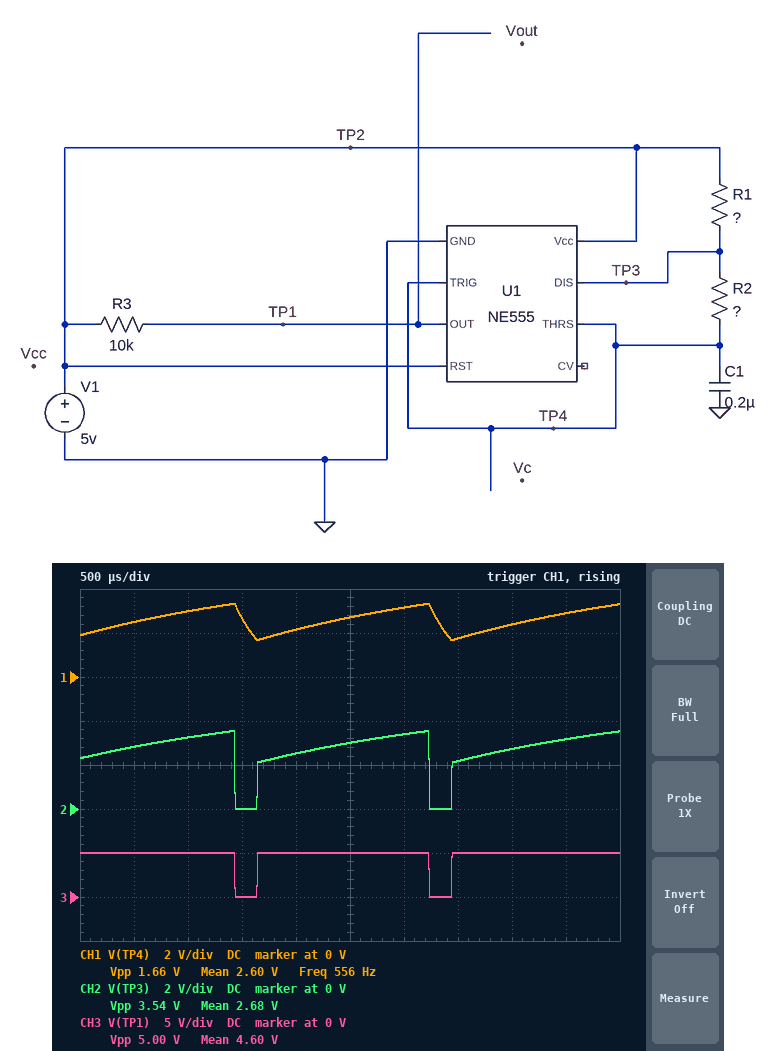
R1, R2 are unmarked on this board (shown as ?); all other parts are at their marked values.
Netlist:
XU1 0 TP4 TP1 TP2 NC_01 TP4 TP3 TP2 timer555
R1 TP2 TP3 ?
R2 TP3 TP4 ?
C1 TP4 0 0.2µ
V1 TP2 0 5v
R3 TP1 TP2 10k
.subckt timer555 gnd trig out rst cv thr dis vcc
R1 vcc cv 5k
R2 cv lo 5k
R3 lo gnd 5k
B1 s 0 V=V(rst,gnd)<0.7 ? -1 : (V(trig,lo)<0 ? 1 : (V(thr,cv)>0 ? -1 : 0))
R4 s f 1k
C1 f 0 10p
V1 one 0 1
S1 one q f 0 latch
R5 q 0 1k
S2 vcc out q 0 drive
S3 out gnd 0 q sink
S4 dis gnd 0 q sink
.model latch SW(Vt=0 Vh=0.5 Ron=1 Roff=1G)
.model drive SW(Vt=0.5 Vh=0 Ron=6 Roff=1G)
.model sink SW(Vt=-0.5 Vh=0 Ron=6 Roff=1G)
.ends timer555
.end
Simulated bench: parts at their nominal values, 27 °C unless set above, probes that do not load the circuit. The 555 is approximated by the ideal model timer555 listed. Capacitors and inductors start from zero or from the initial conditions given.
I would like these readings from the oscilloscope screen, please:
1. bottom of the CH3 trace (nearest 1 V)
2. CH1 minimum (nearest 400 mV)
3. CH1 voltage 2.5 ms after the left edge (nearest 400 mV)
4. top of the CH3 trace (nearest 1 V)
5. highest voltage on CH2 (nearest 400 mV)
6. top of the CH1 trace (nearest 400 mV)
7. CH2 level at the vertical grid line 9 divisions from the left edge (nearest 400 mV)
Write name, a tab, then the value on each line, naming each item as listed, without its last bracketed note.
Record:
bottom of the CH3 trace	0 V
CH1 minimum	1.6 V
CH1 voltage 2.5 ms after the left edge	2.8 V
top of the CH3 trace	5 V
highest voltage on CH2	3.6 V
top of the CH1 trace	3.2 V
CH2 level at the vertical grid line 9 divisions from the left edge	3.2 V
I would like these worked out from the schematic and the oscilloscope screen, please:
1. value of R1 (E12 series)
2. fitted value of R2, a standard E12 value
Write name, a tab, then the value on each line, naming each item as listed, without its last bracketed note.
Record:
value of R1	10 kΩ
fitted value of R2, a standard E12 value	1.5 kΩ
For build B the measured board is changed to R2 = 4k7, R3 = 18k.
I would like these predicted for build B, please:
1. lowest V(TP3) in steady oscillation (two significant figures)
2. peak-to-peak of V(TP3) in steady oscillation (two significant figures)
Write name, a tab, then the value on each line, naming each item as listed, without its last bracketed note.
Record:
lowest V(TP3) in steady oscillation	5.1 mV
peak-to-peak of V(TP3) in steady oscillation	3.9 V
